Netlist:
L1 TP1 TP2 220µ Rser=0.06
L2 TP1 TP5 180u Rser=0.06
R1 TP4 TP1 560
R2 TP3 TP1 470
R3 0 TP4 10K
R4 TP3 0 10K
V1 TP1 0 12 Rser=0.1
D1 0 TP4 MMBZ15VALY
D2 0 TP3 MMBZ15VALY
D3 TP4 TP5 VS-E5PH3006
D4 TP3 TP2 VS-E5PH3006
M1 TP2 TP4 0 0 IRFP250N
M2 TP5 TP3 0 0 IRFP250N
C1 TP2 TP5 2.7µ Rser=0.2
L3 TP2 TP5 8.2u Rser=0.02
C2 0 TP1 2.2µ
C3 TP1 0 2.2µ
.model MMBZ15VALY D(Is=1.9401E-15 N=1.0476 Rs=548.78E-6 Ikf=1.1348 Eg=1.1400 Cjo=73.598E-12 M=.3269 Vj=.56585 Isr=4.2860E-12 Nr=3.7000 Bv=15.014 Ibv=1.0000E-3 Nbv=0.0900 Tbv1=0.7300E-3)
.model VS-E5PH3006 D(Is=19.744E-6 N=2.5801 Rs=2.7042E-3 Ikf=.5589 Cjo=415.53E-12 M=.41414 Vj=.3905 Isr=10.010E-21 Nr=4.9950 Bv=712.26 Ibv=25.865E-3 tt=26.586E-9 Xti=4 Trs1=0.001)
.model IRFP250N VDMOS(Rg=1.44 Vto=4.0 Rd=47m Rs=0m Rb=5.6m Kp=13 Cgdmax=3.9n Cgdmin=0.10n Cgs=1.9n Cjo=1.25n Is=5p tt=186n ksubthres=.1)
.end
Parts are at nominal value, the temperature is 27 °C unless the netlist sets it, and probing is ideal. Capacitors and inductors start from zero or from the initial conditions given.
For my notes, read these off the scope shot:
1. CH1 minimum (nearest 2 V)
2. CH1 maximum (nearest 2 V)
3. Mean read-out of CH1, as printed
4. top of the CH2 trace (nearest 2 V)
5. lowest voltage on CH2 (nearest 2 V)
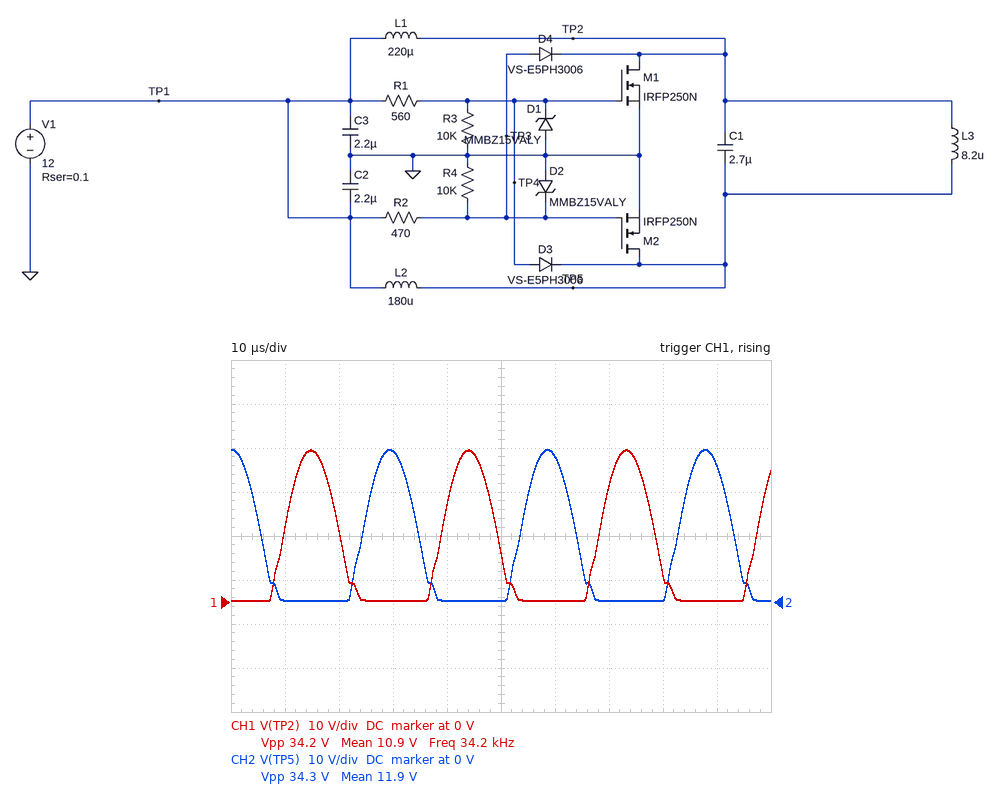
0 V
34 V
10.9 V
34 V
0 V
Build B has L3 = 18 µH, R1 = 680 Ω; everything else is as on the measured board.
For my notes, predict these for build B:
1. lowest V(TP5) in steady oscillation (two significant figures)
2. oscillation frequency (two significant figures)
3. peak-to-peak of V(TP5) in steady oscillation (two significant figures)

100 mV
23 kHz
36 V
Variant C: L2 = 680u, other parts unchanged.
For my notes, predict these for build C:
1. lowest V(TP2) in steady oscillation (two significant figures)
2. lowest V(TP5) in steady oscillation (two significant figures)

230 mV
210 mV
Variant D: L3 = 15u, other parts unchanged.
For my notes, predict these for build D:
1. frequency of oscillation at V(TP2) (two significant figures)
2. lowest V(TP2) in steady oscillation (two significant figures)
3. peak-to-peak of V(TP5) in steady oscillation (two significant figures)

26 kHz
120 mV
36 V
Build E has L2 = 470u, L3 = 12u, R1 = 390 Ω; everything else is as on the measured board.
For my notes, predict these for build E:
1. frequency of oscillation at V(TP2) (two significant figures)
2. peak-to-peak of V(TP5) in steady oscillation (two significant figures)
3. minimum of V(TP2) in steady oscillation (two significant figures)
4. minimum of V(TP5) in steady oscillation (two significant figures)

28 kHz
35 V
160 mV
140 mV
